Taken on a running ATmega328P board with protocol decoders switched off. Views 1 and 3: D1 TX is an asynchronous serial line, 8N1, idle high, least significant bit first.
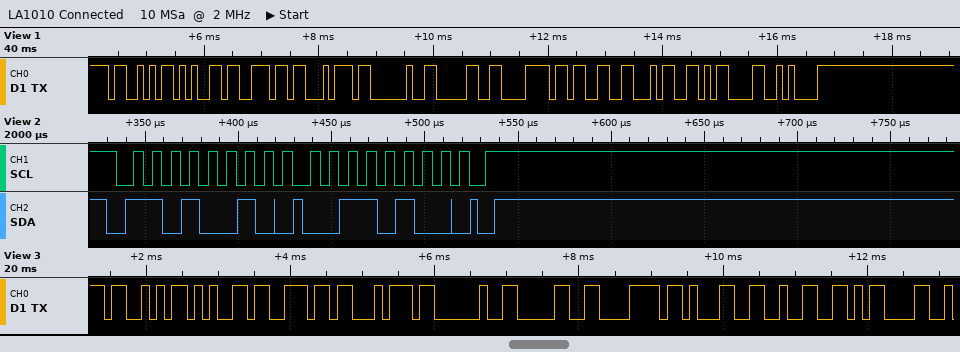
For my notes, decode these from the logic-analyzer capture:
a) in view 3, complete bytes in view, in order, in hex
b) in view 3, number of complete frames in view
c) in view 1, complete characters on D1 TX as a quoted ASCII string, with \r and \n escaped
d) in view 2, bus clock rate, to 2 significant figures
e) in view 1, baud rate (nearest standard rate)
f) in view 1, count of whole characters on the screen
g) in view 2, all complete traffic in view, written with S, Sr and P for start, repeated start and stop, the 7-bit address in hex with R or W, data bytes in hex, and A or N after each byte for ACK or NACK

0x53 0x65 0x6E 0x74 0x20 0x30 0x78 0x31 0x32 0x0D
10
"Sent 0x34\r\n"
100 kHz
9600 baud
11
S 69W A 34 A P
